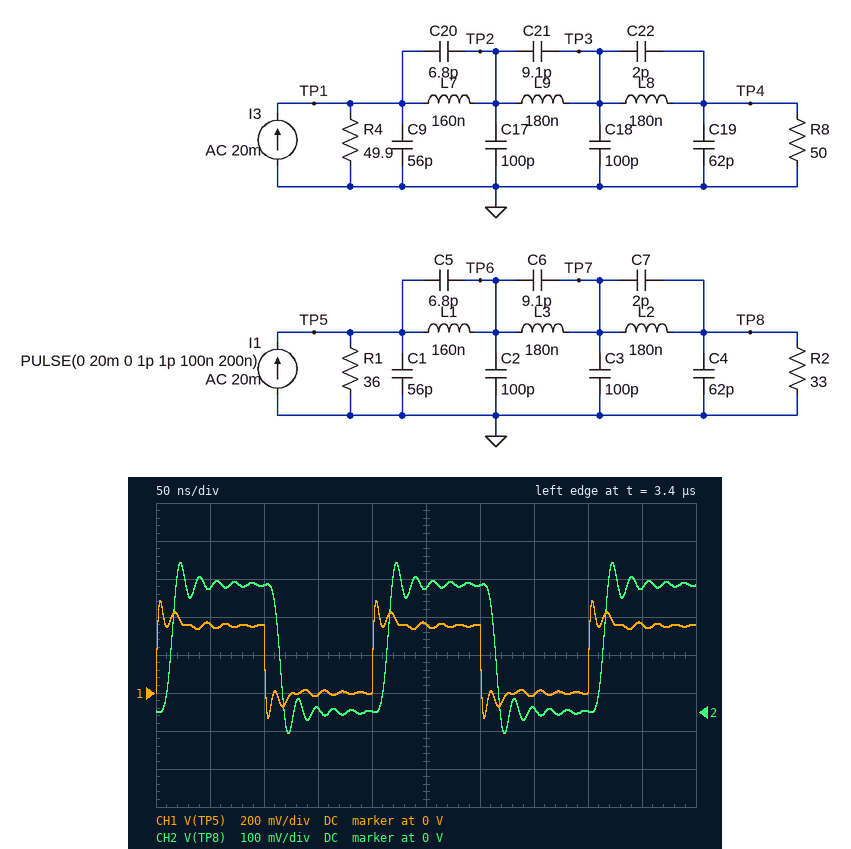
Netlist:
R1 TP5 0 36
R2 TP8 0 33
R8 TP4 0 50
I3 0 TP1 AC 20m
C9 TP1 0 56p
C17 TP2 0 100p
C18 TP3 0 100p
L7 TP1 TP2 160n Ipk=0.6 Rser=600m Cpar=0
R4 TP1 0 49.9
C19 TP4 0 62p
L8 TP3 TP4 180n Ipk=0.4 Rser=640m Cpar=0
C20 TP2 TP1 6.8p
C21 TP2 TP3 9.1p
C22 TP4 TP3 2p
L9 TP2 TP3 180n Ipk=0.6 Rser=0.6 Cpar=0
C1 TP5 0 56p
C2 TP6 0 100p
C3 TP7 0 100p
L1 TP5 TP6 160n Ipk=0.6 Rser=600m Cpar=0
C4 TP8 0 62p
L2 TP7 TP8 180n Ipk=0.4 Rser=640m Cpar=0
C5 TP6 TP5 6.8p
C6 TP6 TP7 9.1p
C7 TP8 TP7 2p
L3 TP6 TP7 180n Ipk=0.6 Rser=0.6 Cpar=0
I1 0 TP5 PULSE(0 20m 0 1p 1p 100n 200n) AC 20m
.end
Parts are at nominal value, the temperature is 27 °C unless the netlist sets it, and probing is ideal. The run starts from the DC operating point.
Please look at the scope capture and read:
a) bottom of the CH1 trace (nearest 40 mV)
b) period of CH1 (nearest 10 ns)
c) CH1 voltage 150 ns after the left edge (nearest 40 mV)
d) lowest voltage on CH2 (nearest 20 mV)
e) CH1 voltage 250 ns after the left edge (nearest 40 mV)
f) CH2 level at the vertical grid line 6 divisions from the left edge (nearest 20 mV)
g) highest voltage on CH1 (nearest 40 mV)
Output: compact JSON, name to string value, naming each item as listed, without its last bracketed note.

{"bottom of the CH1 trace": "-120 mV", "period of CH1": "200 ns", "CH1 voltage 150 ns after the left edge": "0 V", "lowest voltage on CH2": "-60 mV", "CH1 voltage 250 ns after the left edge": "360 mV", "CH2 level at the vertical grid line 6 divisions from the left edge": "340 mV", "highest voltage on CH1": "480 mV"}
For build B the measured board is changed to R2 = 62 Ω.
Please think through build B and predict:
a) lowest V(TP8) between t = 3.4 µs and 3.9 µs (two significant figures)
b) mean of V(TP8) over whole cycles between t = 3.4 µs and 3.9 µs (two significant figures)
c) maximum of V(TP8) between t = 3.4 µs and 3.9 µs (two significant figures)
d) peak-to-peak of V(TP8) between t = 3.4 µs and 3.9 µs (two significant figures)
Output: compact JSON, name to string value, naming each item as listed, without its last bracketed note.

{"lowest V(TP8) between t = 3.4 µs and 3.9 µs": "-92 mV", "mean of V(TP8) over whole cycles between t = 3.4 µs and 3.9 µs": "220 mV", "maximum of V(TP8) between t = 3.4 µs and 3.9 µs": "540 mV", "peak-to-peak of V(TP8) between t = 3.4 µs and 3.9 µs": "630 mV"}
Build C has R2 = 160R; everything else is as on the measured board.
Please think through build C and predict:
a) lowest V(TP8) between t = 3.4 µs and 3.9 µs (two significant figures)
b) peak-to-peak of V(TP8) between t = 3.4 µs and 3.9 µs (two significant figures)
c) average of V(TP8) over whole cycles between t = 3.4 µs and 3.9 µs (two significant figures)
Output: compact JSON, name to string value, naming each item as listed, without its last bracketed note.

{"lowest V(TP8) between t = 3.4 µs and 3.9 µs": "-150 mV", "peak-to-peak of V(TP8) between t = 3.4 µs and 3.9 µs": "890 mV", "average of V(TP8) over whole cycles between t = 3.4 µs and 3.9 µs": "290 mV"}
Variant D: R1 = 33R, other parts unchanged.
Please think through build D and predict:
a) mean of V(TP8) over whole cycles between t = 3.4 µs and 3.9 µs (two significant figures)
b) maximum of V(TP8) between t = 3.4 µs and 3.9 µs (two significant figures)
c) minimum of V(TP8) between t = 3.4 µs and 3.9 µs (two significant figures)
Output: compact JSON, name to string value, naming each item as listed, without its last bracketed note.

{"mean of V(TP8) over whole cycles between t = 3.4 µs and 3.9 µs": "160 mV", "maximum of V(TP8) between t = 3.4 µs and 3.9 µs": "370 mV", "minimum of V(TP8) between t = 3.4 µs and 3.9 µs": "-52 mV"}
